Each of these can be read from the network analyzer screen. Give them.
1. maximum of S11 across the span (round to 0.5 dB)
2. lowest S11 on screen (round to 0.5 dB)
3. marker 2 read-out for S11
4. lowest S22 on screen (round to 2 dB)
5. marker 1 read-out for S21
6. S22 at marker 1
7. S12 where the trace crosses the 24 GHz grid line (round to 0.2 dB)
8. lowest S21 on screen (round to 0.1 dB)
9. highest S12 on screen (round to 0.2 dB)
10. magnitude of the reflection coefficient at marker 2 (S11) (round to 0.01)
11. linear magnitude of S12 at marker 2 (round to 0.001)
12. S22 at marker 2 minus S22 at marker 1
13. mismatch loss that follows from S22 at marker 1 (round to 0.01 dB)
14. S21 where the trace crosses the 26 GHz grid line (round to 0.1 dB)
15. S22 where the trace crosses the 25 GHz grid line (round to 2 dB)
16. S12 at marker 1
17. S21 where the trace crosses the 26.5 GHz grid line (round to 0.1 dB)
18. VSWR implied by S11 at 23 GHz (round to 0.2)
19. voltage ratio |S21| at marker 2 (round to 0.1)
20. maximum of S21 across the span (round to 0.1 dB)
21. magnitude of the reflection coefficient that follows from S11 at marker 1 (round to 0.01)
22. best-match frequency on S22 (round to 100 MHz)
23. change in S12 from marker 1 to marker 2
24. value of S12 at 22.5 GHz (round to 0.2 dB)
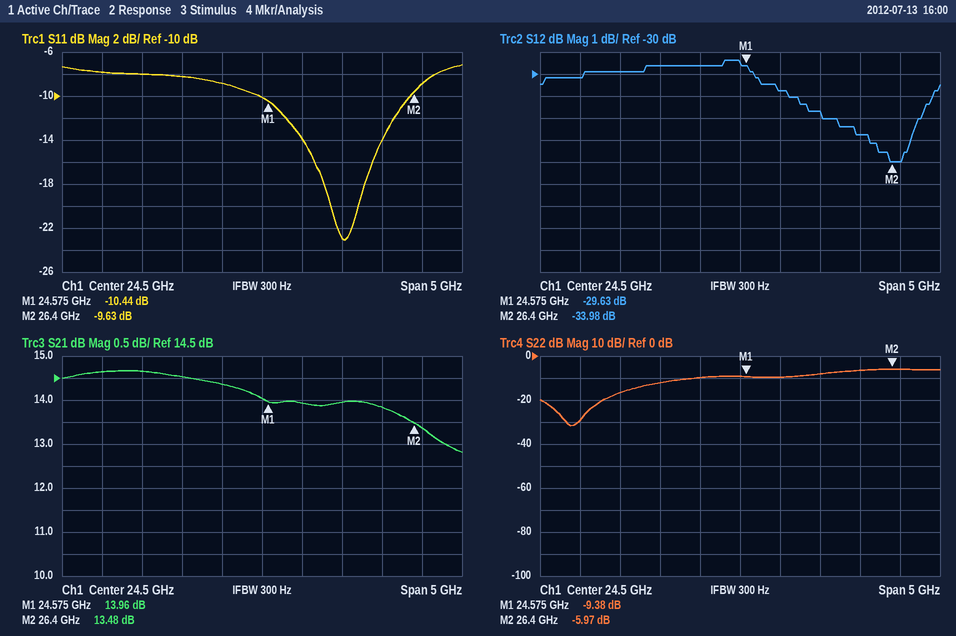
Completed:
-7.0 dB
-23.0 dB
-9.63 dB
-32 dB
13.96 dB
-9.38 dB
-29.6 dB
12.8 dB
-29.4 dB
0.33
0.020
3.41 dB
0.53 dB
13.8 dB
-10 dB
-29.63 dB
13.4 dB
2.4
4.7
14.7 dB
0.30
22.4 GHz
-4.35 dB
-30.2 dB
